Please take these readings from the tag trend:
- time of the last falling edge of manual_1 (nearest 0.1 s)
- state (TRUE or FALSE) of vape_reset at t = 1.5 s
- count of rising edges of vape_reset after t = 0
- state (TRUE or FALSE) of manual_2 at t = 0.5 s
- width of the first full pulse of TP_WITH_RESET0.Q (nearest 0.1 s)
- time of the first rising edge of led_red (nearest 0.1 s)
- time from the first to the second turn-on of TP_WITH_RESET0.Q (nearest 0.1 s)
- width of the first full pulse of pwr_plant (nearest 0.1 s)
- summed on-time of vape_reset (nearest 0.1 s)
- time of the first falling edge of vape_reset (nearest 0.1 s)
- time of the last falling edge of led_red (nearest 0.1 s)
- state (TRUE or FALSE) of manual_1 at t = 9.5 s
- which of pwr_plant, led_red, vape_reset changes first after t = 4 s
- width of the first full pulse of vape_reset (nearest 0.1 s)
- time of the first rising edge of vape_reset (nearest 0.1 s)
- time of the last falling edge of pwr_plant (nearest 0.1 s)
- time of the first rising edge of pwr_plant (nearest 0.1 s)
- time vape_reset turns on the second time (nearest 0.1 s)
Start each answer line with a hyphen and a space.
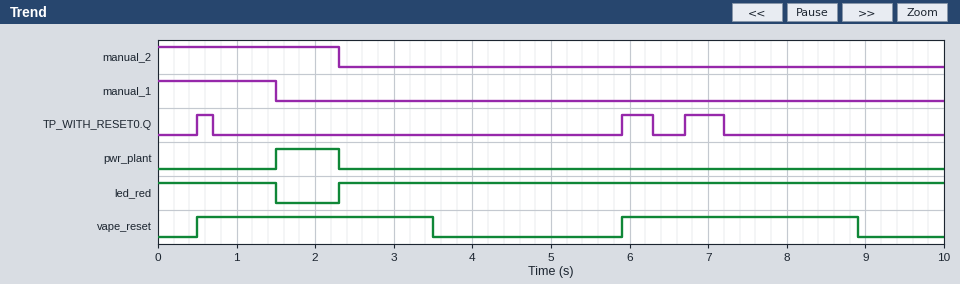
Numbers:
- 1.5 s
- TRUE
- 2
- TRUE
- 0.2 s
- 2.3 s
- 5.4 s
- 0.8 s
- 6.0 s
- 3.5 s
- 1.5 s
- FALSE
- vape_reset
- 3.0 s
- 0.5 s
- 2.3 s
- 1.5 s
- 5.9 s
